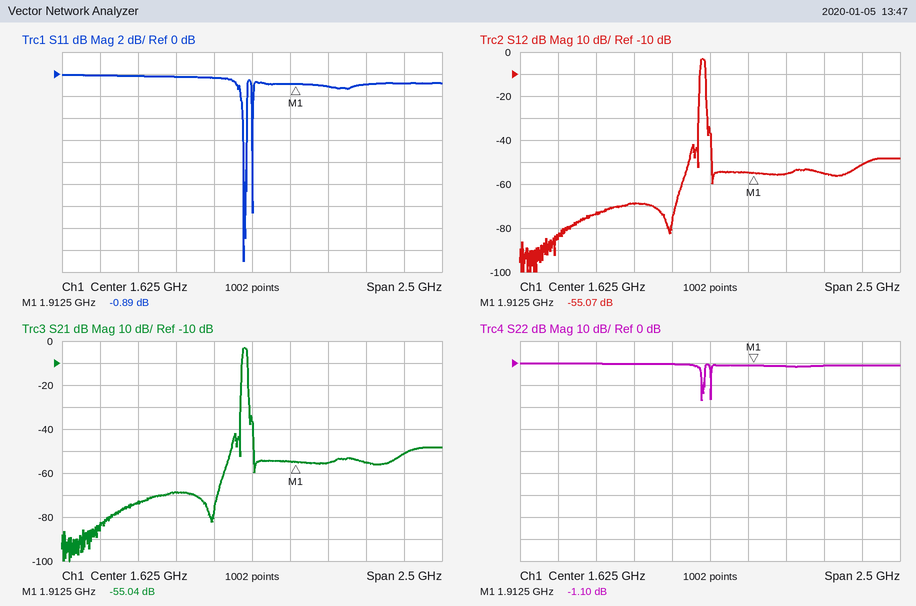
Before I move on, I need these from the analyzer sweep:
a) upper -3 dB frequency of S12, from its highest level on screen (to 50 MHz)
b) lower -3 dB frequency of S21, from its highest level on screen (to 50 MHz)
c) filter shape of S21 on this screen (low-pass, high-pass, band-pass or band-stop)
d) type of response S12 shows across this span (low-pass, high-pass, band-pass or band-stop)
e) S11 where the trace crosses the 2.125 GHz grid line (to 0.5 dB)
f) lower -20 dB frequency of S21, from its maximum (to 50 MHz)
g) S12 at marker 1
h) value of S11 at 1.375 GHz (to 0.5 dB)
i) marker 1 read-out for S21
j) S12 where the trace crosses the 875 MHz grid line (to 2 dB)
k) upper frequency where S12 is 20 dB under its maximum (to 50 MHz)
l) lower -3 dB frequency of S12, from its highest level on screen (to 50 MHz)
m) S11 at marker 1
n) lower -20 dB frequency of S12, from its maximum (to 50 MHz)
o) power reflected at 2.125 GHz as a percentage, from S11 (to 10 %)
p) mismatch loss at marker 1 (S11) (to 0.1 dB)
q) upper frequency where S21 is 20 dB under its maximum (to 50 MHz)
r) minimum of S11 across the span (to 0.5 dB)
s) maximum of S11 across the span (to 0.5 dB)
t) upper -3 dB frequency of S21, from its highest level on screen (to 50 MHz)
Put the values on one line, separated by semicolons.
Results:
1.60 GHz; 1.55 GHz; band-pass; band-pass; -1.0 dB; 1.55 GHz; -55.07 dB; -0.5 dB; -55.04 dB; -74 dB; 1.60 GHz; 1.55 GHz; -0.89 dB; 1.55 GHz; 80 %; 7.3 dB; 1.60 GHz; -17.0 dB; 0.0 dB; 1.60 GHz
